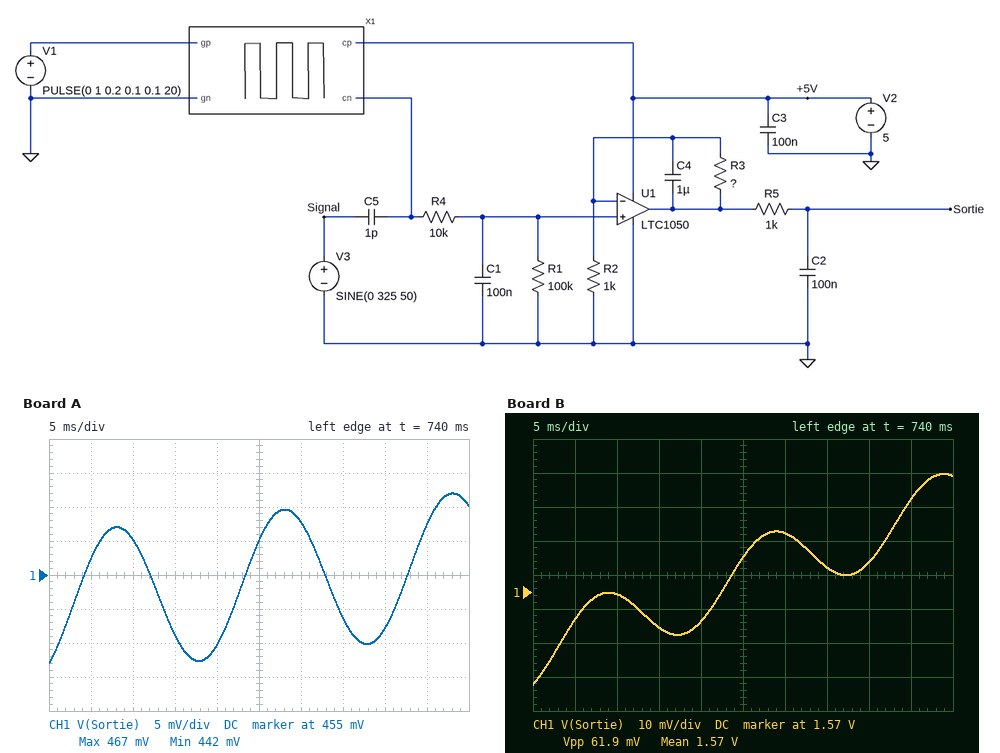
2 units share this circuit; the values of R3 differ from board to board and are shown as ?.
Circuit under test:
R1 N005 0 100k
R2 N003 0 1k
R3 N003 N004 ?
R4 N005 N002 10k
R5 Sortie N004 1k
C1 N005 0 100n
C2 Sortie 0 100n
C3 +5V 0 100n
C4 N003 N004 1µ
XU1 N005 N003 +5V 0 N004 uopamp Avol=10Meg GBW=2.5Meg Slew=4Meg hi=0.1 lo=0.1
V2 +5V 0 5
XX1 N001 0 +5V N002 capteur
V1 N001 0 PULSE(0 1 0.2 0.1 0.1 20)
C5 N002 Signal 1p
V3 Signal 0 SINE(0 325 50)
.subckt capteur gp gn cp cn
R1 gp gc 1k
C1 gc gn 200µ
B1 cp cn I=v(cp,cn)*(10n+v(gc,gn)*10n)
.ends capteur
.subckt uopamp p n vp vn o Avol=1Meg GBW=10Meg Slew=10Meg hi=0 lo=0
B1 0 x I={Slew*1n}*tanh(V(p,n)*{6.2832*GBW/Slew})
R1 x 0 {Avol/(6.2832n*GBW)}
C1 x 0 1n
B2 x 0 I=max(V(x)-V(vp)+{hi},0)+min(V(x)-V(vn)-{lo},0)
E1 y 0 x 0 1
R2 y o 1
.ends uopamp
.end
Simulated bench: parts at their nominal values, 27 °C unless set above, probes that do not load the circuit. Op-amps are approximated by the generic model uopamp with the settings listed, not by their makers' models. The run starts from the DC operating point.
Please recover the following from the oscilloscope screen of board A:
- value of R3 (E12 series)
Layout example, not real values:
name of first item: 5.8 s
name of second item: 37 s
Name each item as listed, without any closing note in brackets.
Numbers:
value of R3: 47 kΩ
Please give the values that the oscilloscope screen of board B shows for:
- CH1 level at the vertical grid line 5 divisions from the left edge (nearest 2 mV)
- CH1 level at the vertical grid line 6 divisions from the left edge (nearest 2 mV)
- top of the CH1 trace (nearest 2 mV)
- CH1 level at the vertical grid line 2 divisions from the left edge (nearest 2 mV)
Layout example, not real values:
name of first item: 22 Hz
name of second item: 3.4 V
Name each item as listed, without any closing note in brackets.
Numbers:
CH1 level at the vertical grid line 5 divisions from the left edge: 1.580 V
CH1 level at the vertical grid line 6 divisions from the left edge: 1.588 V
top of the CH1 trace: 1.604 V
CH1 level at the vertical grid line 2 divisions from the left edge: 1.570 V
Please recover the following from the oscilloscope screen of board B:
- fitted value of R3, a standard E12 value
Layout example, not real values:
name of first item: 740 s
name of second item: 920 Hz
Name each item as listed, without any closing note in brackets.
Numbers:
fitted value of R3, a standard E12 value: 180 kΩ
